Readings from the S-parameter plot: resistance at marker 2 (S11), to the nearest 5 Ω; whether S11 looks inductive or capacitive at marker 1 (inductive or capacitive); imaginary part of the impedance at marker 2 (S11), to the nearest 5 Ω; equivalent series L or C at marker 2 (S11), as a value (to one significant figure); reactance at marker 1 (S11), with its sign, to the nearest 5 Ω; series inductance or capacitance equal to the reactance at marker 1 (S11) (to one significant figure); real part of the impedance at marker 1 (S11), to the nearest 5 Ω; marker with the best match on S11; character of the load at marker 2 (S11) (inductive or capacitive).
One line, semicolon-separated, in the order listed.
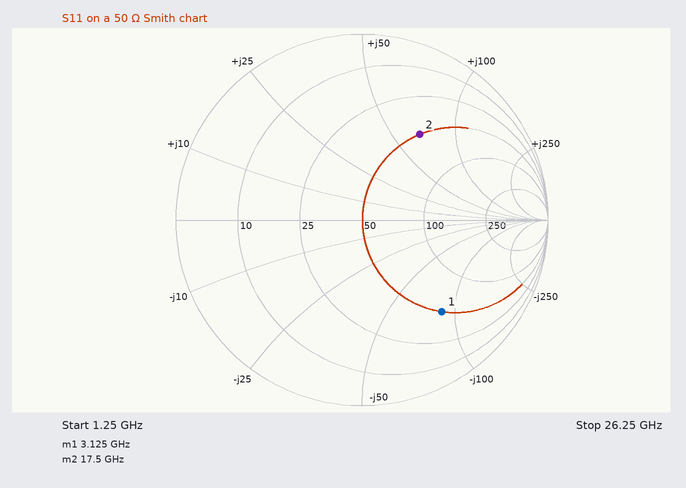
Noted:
50 Ω; capacitive; +65 Ω; 600 pH; -85 Ω; 600 fF; 50 Ω; marker 2; inductive
